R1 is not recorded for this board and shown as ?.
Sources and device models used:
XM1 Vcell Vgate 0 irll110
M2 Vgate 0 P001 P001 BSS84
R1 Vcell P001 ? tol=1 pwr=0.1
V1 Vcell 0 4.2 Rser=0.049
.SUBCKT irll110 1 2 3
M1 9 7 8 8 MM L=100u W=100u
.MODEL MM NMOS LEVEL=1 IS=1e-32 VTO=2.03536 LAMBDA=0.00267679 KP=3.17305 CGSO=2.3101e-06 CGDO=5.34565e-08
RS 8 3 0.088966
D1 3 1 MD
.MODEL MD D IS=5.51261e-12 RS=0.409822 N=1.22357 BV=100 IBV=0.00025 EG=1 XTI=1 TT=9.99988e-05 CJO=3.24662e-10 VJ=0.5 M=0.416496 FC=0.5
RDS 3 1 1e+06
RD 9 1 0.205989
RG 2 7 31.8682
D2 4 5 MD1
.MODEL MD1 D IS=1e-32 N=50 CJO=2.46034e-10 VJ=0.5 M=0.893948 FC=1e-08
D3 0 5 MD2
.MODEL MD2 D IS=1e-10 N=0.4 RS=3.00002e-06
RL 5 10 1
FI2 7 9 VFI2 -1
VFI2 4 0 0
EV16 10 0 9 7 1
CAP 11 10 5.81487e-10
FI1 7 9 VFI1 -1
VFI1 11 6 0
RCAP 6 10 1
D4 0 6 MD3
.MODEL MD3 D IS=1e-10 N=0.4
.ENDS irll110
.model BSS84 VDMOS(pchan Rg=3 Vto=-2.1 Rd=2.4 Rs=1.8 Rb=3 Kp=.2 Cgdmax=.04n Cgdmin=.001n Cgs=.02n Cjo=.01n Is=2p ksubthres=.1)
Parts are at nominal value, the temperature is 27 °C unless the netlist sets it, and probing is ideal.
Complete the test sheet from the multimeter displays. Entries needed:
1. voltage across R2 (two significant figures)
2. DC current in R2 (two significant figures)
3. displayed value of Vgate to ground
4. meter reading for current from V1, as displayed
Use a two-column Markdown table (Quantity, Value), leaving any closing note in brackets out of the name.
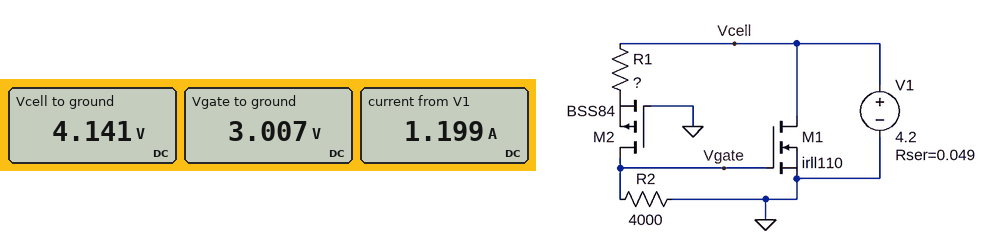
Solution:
| Quantity | Value |
|---|---|
| voltage across R2 | 3.0 V |
| DC current in R2 | 750 µA |
| displayed value of Vgate to ground | 3.007 V |
| meter reading for current from V1, as displayed | 1.199 A |
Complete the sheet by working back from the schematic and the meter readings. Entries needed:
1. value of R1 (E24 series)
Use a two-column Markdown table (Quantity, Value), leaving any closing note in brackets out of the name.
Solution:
| Quantity | Value |
|---|---|
| value of R1 | 1.5 kΩ |
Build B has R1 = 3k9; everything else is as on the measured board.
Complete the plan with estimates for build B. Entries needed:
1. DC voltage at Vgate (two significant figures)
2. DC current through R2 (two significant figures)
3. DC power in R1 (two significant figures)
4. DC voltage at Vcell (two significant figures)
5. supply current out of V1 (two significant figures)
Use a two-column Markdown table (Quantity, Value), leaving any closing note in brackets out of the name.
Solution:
| Quantity | Value |
|---|---|
| DC voltage at Vgate | 2.1 V |
| DC current through R2 | 530 µA |
| DC power in R1 | 1.1 mW |
| DC voltage at Vcell | 4.2 V |
| supply current out of V1 | 8.8 mA |
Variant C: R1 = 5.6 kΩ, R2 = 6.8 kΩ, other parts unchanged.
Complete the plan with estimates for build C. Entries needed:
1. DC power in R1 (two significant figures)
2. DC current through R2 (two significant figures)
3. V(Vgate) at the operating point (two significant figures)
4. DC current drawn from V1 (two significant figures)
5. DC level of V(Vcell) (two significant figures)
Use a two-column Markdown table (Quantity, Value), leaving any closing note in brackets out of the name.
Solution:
| Quantity | Value |
|---|---|
| DC power in R1 | 640 µW |
| DC current through R2 | 340 µA |
| V(Vgate) at the operating point | 2.3 V |
| DC current drawn from V1 | 100 mA |
| DC level of V(Vcell) | 4.2 V |
